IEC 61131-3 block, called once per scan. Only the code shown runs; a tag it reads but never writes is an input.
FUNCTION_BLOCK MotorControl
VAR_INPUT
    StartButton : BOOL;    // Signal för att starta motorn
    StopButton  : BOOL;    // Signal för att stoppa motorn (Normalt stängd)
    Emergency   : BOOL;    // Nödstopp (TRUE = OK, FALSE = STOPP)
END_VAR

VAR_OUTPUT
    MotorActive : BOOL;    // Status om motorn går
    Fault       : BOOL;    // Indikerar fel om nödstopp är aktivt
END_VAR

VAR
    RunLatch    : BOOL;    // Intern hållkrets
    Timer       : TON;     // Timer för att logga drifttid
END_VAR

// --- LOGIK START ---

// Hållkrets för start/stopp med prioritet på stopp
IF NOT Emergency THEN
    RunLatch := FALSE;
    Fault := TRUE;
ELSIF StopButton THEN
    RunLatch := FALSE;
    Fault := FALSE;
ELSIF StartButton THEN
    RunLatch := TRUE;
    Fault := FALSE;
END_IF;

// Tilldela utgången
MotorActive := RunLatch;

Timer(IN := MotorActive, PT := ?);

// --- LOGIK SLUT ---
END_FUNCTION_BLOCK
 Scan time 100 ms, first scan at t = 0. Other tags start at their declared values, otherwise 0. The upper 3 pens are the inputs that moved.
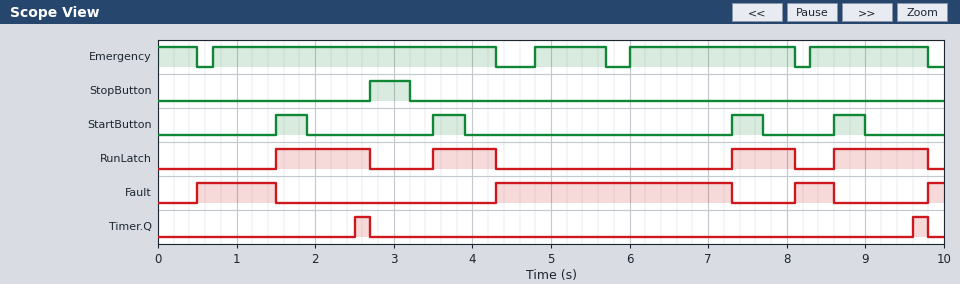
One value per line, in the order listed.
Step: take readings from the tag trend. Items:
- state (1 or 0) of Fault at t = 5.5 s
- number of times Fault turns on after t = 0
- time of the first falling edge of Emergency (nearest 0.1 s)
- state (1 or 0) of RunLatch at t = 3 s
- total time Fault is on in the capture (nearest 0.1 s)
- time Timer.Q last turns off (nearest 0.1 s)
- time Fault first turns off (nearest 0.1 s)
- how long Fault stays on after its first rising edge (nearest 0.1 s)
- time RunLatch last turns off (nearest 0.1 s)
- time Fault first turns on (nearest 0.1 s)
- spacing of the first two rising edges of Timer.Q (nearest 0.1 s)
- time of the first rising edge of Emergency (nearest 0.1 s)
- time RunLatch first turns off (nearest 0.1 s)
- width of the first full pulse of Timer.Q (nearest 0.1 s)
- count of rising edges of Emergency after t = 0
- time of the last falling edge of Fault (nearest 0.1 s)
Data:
1
4
0.5 s
0
4.7 s
9.8 s
1.5 s
1.0 s
9.8 s
0.5 s
7.1 s
0.7 s
2.7 s
0.2 s
4
8.6 s
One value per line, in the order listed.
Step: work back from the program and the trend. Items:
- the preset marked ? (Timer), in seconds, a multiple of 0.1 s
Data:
1.0 s
